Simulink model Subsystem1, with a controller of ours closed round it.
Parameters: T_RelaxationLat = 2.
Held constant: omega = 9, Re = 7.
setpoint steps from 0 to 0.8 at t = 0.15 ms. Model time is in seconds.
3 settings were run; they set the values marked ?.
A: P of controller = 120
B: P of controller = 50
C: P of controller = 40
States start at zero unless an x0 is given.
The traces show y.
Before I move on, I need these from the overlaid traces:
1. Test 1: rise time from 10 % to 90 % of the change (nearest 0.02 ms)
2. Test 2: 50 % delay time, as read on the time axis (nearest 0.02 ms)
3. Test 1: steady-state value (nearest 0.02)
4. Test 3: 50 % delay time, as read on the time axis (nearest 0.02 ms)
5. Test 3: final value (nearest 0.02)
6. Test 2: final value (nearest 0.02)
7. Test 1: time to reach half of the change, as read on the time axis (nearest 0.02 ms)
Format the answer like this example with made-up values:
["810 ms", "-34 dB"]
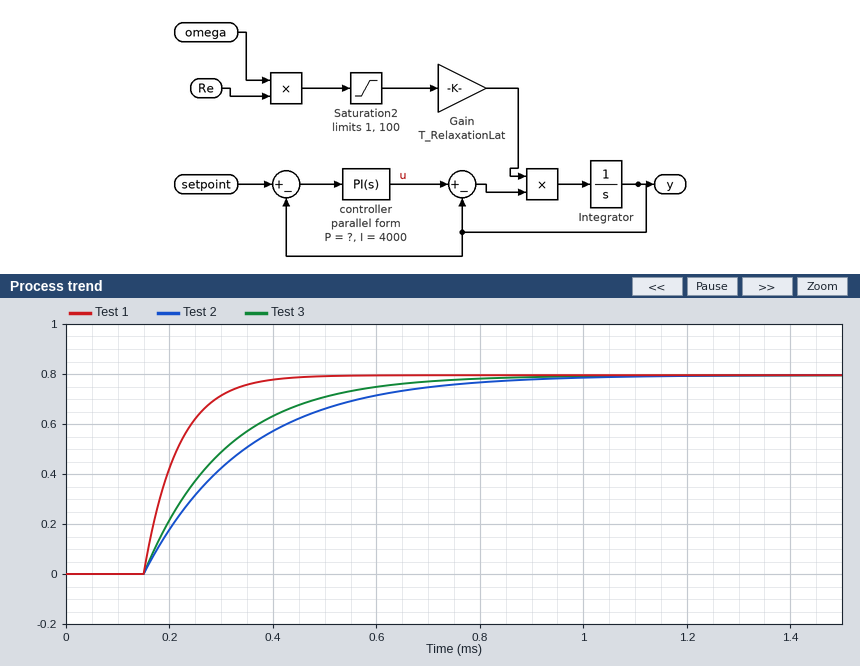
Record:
["0.14 ms", "0.28 ms", "0.80", "0.26 ms", "0.80", "0.80", "0.20 ms"]
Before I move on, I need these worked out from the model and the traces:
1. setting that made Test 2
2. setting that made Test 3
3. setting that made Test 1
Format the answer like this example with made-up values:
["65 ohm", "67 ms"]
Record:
["C", "B", "A"]
